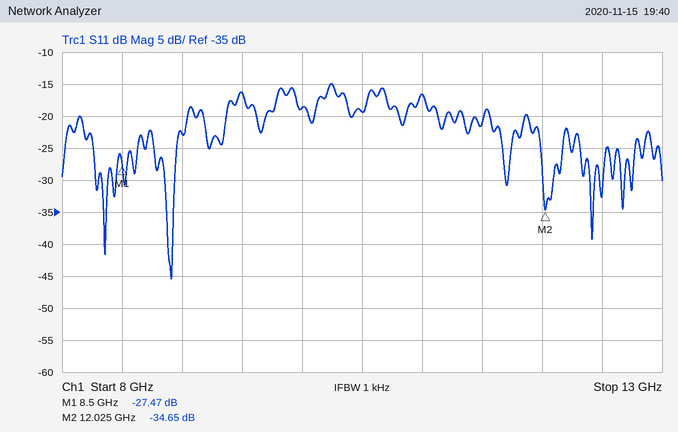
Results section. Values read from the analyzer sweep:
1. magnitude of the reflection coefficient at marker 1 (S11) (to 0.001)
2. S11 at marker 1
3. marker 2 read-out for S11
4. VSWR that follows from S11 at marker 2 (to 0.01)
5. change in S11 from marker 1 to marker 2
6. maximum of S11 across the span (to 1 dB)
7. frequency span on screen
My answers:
0.042
-27.47 dB
-34.65 dB
1.04
-7.18 dB
-15 dB
5 GHz
